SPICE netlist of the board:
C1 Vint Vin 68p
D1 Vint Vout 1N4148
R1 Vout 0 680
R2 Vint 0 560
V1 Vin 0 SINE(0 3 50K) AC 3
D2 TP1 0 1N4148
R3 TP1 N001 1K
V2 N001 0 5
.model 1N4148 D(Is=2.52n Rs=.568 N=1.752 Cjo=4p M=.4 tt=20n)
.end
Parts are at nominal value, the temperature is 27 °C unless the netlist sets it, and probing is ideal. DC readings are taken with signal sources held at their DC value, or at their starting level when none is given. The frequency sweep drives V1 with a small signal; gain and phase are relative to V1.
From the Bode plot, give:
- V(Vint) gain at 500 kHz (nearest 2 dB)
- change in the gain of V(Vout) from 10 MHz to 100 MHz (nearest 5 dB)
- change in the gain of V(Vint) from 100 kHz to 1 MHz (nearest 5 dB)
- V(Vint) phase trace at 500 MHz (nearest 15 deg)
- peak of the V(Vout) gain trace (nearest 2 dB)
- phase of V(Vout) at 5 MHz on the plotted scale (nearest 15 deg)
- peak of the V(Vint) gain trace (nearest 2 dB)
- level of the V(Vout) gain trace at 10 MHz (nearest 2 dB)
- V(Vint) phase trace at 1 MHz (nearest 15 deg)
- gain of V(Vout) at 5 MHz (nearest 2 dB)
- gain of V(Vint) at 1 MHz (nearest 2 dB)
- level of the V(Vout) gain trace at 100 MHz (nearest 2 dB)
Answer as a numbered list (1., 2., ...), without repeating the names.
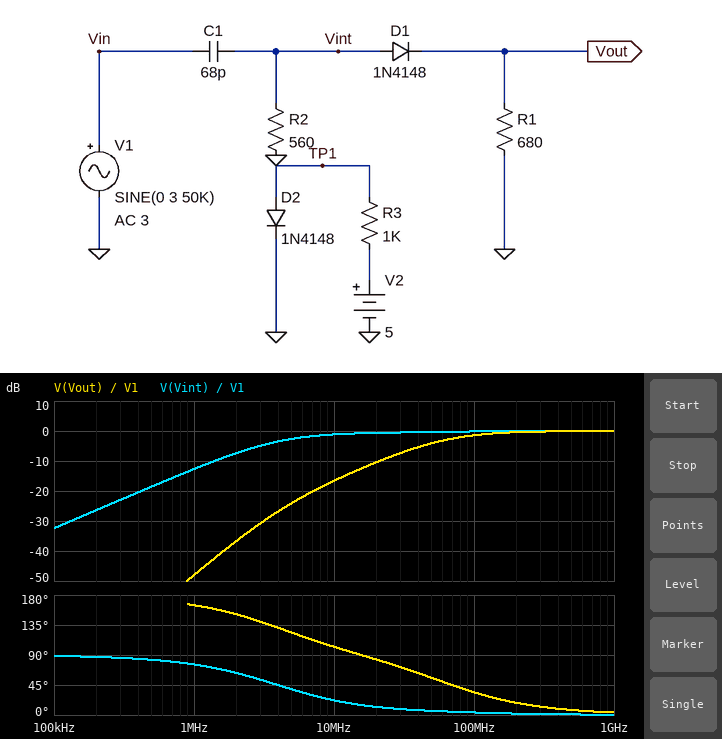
1. -18 dB
2. 15 dB
3. 20 dB
4. 0 deg
5. 0 dB
6. 120 deg
7. 0 dB
8. -16 dB
9. 75 deg
10. -24 dB
11. -12 dB
12. -2 dB
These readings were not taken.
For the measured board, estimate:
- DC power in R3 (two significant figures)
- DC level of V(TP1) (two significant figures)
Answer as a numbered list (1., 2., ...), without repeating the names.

1. 19 mW
2. 650 mV
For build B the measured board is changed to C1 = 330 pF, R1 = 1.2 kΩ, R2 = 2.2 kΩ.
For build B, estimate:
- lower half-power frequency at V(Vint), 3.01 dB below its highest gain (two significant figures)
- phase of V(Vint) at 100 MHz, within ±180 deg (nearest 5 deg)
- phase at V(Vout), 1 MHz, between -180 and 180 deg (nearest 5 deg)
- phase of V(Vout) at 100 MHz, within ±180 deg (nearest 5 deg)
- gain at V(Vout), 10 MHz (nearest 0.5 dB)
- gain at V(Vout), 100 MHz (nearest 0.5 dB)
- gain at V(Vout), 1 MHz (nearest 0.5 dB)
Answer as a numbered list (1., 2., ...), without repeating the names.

1. 220 kHz
2. 0 deg
3. 100 deg
4. 20 deg
5. -11.0 dB
6. -0.5 dB
7. -30.5 dB
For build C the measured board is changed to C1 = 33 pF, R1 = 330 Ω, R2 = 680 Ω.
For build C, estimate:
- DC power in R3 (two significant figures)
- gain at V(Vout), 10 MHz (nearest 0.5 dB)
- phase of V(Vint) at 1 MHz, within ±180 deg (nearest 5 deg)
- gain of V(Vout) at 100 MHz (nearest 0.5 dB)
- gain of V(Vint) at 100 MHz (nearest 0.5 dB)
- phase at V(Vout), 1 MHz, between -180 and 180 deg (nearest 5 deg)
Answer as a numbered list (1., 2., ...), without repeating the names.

1. 19 mW
2. -24.0 dB
3. 80 deg
4. -4.5 dB
5. -0.5 dB
6. 170 deg
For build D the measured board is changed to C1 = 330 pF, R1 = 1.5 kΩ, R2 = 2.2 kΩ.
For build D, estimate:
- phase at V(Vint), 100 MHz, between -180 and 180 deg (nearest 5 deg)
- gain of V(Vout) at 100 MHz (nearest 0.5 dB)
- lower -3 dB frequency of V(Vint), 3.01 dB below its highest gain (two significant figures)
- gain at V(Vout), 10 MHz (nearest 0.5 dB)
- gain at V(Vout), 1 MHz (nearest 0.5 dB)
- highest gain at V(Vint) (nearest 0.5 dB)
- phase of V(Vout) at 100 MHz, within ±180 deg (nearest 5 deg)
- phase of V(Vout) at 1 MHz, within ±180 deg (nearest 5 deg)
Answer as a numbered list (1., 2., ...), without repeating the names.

1. 0 deg
2. -0.5 dB
3. 220 kHz
4. -9.0 dB
5. -29.0 dB
6. 0 dB
7. 15 deg
8. 100 deg
